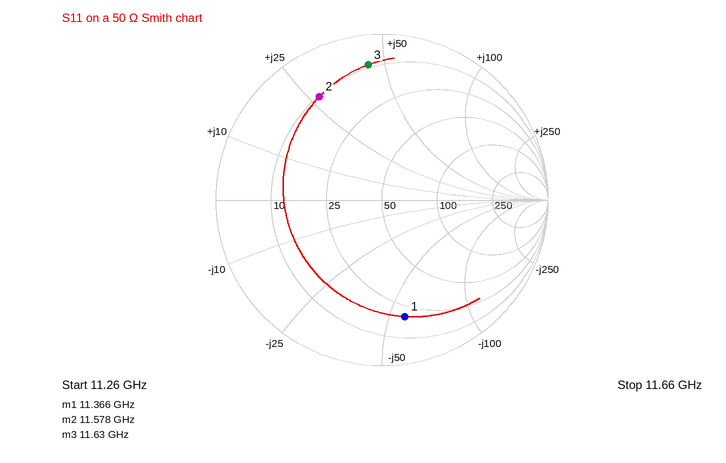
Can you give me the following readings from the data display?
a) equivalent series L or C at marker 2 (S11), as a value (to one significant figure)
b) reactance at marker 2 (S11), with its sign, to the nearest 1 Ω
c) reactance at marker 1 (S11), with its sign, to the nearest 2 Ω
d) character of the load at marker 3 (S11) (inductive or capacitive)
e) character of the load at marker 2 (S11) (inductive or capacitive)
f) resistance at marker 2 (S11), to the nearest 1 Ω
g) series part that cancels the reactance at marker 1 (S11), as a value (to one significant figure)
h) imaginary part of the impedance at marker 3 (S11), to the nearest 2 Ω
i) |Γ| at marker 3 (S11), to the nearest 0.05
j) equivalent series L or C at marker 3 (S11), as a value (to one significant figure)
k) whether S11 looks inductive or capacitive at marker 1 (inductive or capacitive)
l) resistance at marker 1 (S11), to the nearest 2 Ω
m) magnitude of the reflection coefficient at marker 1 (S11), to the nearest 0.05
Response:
400 pH
+27 Ω
-56 Ω
inductive
inductive
10 Ω
800 pH
+44 Ω
0.80
600 pH
capacitive
20 Ω
0.70
